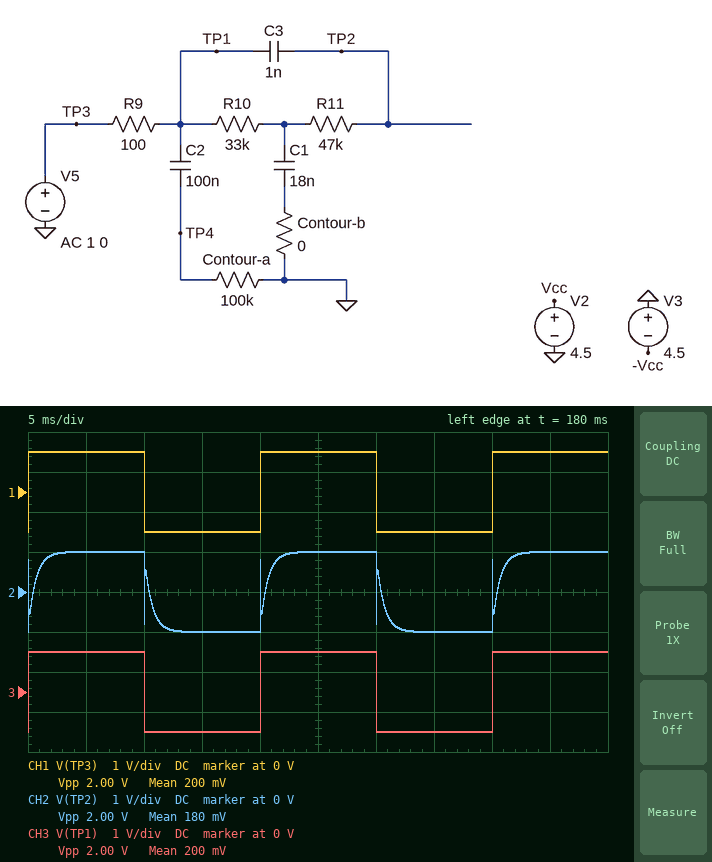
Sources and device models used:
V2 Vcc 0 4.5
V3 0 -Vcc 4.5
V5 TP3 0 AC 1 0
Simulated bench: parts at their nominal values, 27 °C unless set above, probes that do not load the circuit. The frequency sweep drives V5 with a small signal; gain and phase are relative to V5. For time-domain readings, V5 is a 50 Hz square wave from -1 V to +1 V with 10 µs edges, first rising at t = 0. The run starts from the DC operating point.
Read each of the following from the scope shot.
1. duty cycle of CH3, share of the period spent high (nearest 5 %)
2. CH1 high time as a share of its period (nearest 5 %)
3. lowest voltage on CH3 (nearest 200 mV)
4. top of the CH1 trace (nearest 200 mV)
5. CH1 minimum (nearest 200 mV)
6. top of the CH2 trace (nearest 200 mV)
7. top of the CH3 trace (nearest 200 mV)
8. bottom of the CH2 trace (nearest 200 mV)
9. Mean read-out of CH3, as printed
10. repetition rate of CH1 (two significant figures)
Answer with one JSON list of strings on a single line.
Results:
["50 %", "50 %", "-1.0 V", "1.0 V", "-1.0 V", "1.0 V", "1.0 V", "-1.0 V", "200 mV", "50 Hz"]
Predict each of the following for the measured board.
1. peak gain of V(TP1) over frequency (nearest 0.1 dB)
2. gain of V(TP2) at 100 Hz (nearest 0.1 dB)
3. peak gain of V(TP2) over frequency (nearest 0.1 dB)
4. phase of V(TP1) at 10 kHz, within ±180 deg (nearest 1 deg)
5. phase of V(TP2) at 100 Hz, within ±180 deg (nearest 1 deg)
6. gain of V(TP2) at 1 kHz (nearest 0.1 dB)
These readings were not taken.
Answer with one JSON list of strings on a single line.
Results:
["0 dB", "-0.7 dB", "0 dB", "0 deg", "-20 deg", "-18.4 dB"]
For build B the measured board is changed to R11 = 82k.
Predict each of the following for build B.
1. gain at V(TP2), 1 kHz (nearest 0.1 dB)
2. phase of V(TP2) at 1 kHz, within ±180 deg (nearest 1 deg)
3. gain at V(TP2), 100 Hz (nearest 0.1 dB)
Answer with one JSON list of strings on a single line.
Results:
["-11.8 dB", "40 deg", "-0.8 dB"]
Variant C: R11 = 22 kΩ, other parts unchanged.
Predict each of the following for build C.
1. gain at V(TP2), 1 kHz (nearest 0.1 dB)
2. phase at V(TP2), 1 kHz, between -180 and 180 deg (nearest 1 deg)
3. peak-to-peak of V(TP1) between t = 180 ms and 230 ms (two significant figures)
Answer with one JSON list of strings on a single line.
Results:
["-16.8 dB", "-48 deg", "2.0 V"]
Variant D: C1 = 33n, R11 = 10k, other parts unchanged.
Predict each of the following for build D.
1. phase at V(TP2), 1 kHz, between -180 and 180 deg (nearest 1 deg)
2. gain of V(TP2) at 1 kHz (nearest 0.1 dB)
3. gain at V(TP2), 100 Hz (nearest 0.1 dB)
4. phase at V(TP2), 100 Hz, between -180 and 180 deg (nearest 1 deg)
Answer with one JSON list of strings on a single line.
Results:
["-60 deg", "-21.1 dB", "-1.8 dB", "-34 deg"]
